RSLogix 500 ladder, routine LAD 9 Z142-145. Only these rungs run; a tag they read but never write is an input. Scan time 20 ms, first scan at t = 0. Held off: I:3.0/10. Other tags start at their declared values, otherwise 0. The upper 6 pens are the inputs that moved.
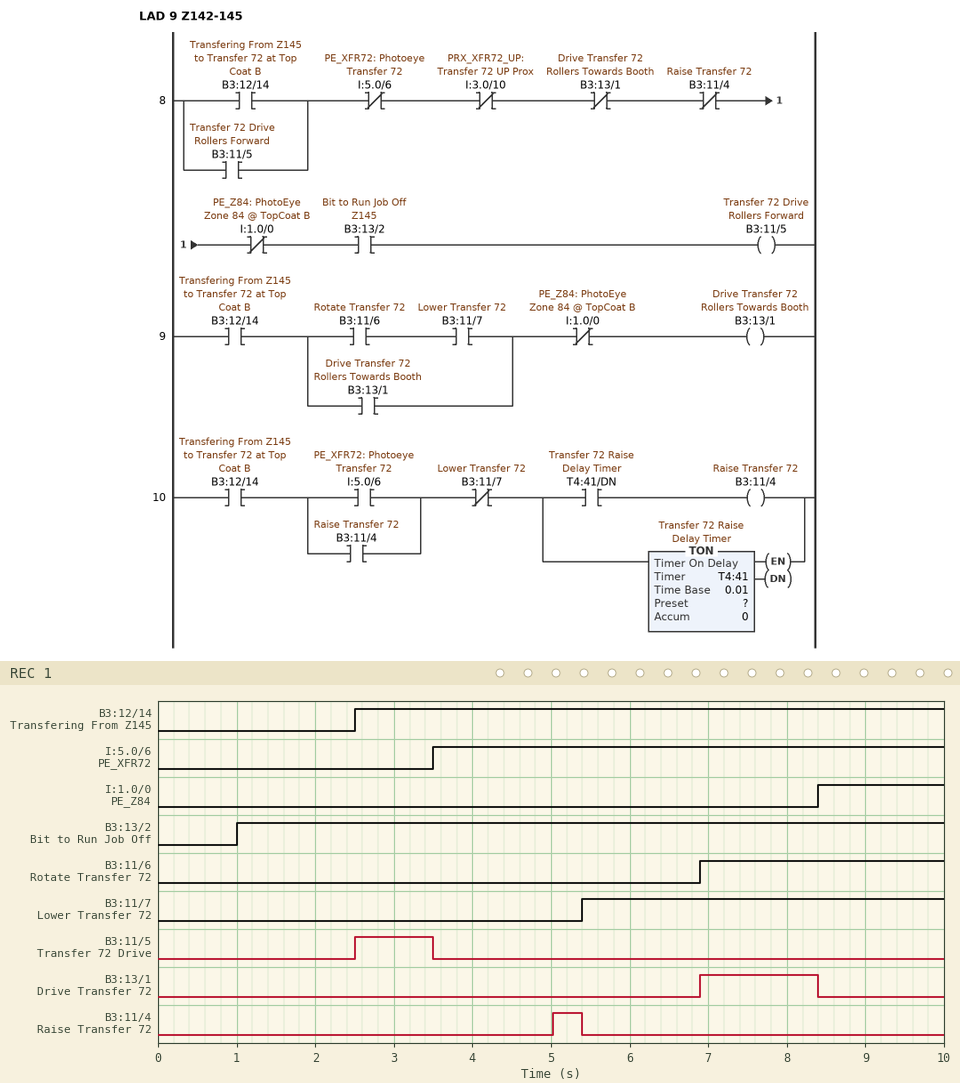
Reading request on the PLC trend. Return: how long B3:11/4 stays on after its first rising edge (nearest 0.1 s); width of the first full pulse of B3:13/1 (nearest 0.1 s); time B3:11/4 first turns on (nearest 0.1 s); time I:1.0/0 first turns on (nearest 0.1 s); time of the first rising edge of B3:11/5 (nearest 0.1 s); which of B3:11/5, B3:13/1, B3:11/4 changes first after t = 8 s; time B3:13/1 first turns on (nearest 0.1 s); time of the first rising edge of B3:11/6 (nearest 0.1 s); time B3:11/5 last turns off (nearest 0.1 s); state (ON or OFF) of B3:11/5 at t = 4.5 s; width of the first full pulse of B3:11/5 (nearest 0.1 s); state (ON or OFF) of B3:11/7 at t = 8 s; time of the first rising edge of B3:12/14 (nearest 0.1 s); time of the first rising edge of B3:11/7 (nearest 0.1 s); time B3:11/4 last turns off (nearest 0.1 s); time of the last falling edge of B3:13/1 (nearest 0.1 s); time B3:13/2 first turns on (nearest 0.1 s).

0.4 s
1.5 s
5.0 s
8.4 s
2.5 s
B3:13/1
6.9 s
6.9 s
3.5 s
OFF
1.0 s
ON
2.5 s
5.4 s
5.4 s
8.4 s
1.0 s
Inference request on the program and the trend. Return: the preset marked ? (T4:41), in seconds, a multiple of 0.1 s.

1.5 s
